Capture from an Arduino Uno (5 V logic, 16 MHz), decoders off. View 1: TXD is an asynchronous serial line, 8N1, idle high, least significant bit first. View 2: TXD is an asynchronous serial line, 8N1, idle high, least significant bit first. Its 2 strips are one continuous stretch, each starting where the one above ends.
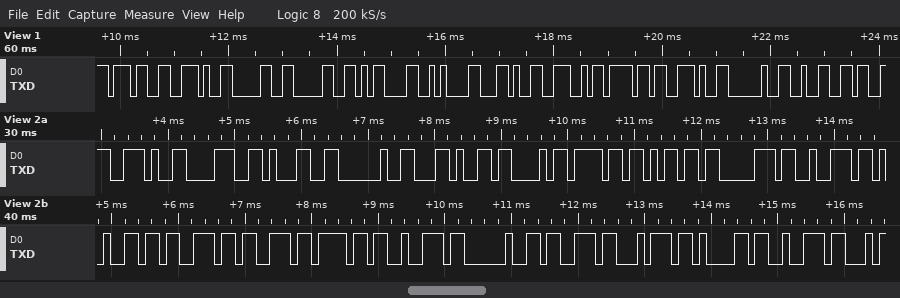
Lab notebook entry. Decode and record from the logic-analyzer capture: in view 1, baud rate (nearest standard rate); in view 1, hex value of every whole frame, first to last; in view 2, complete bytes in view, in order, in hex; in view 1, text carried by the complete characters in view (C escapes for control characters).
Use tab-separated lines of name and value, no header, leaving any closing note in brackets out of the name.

in view 1, baud rate	9600 baud
in view 1, hex value of every whole frame, first to last	37 2E 30 30 0D 0A 2C 4E 6F 2E 20 32
in view 2, complete bytes in view, in order, in hex	2E 38 31 20 2C 43 6F 6D 70 72 65 73 73 6F 72 20 73 74 61 72
in view 1, text carried by the complete characters in view	"7.00\r\n,No. 2"
